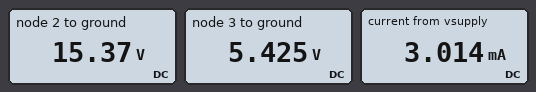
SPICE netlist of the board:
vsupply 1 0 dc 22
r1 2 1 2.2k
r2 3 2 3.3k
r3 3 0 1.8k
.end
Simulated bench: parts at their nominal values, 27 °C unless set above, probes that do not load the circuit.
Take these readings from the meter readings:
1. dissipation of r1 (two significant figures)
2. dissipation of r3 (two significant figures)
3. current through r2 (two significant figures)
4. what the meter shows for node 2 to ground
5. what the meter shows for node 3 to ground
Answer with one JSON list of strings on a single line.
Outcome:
["20 mW", "16 mW", "3.0 mA", "15.37 V", "5.425 V"]
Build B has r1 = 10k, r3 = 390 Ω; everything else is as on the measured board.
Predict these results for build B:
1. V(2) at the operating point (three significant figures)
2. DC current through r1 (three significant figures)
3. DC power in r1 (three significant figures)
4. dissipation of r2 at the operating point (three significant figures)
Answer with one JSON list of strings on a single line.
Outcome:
["5.93 V", "1.61 mA", "25.8 mW", "8.52 mW"]
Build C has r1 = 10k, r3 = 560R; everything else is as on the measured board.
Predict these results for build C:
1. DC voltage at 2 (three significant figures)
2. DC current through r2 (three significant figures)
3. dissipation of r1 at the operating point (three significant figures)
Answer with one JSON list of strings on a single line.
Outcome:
["6.13 V", "1.59 mA", "25.2 mW"]
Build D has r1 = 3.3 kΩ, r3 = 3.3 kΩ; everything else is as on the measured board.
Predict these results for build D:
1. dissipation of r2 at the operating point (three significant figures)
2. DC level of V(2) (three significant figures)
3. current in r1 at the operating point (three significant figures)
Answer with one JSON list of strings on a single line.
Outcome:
["16.3 mW", "14.7 V", "2.22 mA"]
